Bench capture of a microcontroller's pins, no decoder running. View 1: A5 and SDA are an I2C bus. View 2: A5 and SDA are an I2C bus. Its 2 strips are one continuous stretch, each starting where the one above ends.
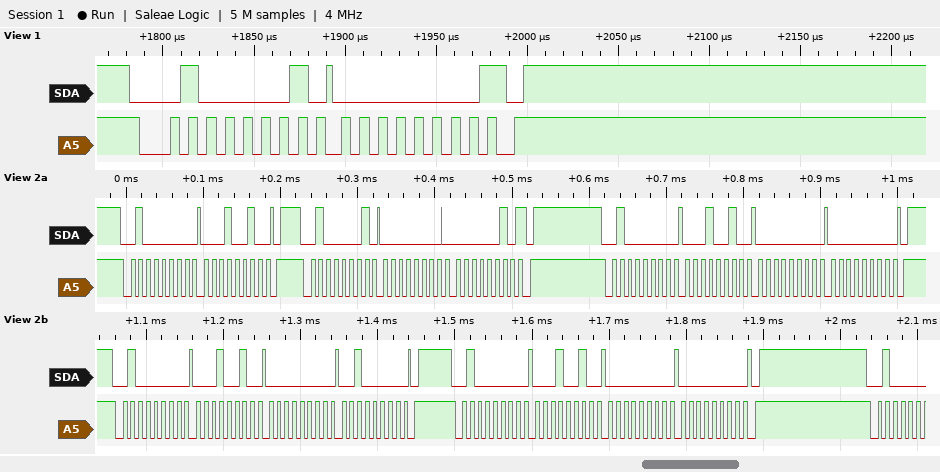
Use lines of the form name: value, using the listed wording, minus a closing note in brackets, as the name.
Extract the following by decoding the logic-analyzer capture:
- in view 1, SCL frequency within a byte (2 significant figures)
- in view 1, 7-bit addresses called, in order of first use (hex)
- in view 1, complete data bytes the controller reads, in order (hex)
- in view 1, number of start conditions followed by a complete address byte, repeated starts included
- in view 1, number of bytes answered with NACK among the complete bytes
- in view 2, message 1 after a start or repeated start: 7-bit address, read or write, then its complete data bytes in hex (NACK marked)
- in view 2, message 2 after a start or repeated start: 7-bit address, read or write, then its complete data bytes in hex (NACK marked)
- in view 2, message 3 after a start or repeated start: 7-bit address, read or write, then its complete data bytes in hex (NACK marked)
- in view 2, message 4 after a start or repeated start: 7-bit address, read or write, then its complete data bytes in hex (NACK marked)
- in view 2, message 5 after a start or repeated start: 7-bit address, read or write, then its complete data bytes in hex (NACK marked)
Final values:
in view 1, SCL frequency within a byte: 100 kHz
in view 1, 7-bit addresses called, in order of first use: 0x20
in view 1, complete data bytes the controller reads, in order: 00
in view 1, number of start conditions followed by a complete address byte, repeated starts included: 1
in view 1, number of bytes answered with NACK among the complete bytes: 1
in view 2, message 1 after a start or repeated start: 7-bit address, read or write, then its complete data bytes in hex: 0x20 write: 12
in view 2, message 2 after a start or repeated start: 7-bit address, read or write, then its complete data bytes in hex: 0x20 read: 00 02 NACK
in view 2, message 3 after a start or repeated start: 7-bit address, read or write, then its complete data bytes in hex: 0x20 write: 12 00 00
in view 2, message 4 after a start or repeated start: 7-bit address, read or write, then its complete data bytes in hex: 0x20 write: 12 00 20
in view 2, message 5 after a start or repeated start: 7-bit address, read or write, then its complete data bytes in hex: 0x20 write: 12 00 00
